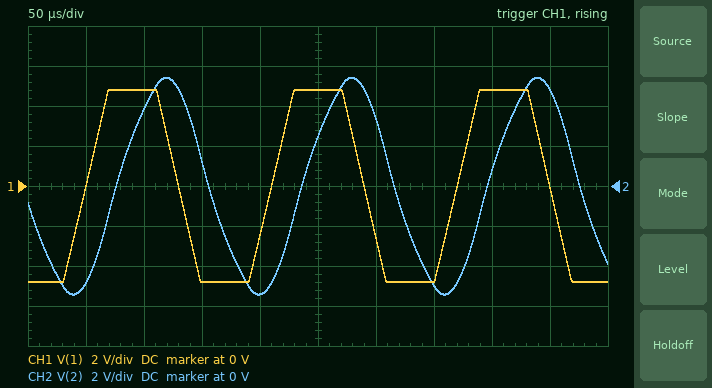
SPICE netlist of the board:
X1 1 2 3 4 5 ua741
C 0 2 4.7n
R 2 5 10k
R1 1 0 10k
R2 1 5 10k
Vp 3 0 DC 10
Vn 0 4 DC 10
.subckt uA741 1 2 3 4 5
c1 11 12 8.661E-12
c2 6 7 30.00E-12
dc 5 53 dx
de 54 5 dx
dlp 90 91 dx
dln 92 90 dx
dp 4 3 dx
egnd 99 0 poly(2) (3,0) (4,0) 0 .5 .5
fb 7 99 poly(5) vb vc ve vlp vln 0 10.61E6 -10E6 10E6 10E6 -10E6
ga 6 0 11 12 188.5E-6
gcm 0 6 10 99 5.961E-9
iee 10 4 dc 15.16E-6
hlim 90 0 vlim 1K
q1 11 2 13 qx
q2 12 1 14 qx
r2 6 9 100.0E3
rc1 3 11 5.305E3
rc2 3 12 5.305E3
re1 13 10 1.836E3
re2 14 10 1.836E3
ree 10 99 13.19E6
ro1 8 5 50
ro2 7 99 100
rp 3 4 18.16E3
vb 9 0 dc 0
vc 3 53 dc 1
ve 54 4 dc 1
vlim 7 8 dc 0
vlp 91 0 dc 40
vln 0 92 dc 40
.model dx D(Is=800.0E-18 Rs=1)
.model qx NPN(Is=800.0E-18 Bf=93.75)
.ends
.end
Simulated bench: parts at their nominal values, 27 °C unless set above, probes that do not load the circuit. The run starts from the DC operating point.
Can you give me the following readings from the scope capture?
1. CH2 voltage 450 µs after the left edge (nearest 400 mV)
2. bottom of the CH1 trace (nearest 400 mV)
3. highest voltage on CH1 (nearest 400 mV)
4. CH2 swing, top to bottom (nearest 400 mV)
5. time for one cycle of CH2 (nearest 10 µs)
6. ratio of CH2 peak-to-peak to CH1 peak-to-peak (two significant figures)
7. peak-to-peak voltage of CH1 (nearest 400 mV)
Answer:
4.8 V
-4.8 V
4.8 V
10.8 V
160 µs
1.1
9.6 V
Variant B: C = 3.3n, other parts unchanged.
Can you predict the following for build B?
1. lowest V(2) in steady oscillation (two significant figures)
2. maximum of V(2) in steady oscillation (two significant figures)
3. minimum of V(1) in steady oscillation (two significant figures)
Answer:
-5.6 V
5.6 V
-4.8 V
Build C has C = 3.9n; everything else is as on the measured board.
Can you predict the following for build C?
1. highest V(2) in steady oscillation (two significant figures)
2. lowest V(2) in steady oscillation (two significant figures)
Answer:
5.5 V
-5.5 V
